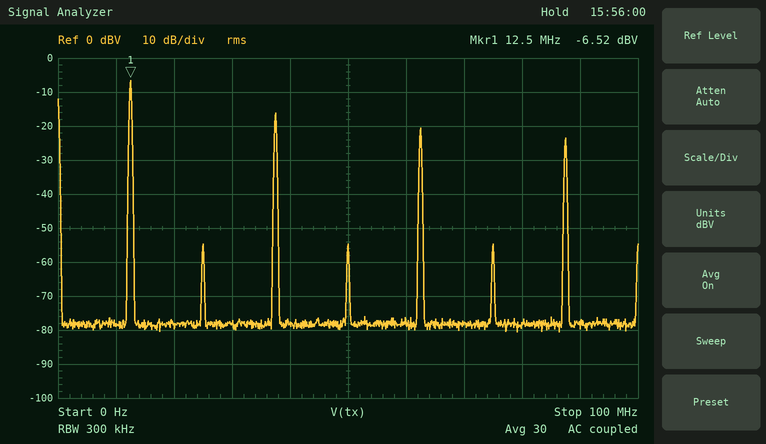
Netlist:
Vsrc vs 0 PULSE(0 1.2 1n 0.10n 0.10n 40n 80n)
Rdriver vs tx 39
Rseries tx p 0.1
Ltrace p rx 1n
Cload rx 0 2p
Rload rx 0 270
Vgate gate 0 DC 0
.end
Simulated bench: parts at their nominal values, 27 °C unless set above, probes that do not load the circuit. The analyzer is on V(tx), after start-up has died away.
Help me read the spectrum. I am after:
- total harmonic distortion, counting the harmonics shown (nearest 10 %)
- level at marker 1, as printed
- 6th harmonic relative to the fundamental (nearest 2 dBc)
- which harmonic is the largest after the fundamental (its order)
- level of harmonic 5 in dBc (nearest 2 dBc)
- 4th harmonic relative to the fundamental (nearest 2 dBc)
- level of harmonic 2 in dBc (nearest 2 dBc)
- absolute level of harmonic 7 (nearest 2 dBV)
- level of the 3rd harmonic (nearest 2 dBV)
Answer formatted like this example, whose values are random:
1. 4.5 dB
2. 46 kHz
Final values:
1. 40 %
2. -6.52 dBV
3. -48 dBc
4. 3
5. -14 dBc
6. -48 dBc
7. -48 dBc
8. -24 dBV
9. -16 dBV
